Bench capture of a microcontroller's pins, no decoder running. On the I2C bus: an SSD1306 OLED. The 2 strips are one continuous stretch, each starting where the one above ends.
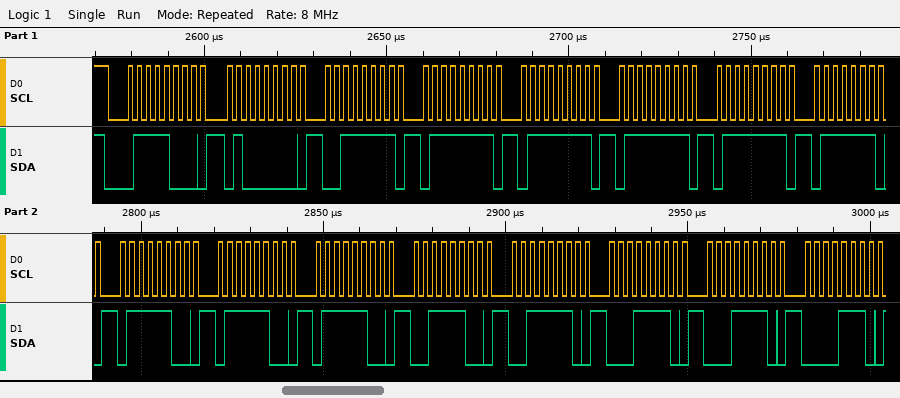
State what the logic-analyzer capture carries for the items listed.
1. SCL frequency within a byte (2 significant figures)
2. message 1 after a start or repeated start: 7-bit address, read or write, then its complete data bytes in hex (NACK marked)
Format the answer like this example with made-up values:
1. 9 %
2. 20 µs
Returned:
1. 400 kHz
2. 0x3C write: 40 3F 7F 7F 7F 7F 7E 7C 7C 7C 3C 3E 1E 1E 0E
